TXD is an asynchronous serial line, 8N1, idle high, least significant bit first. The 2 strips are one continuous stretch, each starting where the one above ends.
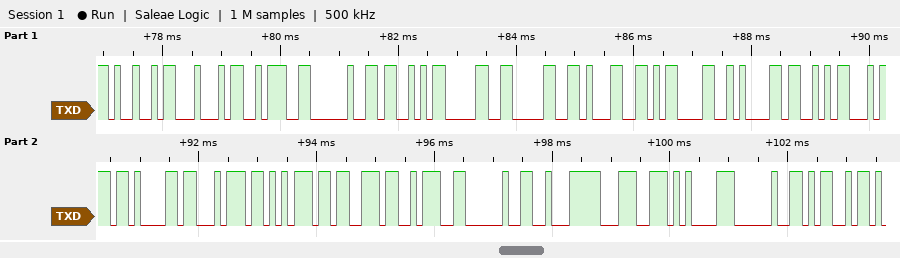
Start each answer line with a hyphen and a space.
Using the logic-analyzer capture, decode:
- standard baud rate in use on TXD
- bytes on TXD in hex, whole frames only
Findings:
- 9600 baud
- 49 44 3A 20 53 30 30 31 0D 0A 53 74 61 74 75 73 3A 20 E2 9C 85 20 4D
